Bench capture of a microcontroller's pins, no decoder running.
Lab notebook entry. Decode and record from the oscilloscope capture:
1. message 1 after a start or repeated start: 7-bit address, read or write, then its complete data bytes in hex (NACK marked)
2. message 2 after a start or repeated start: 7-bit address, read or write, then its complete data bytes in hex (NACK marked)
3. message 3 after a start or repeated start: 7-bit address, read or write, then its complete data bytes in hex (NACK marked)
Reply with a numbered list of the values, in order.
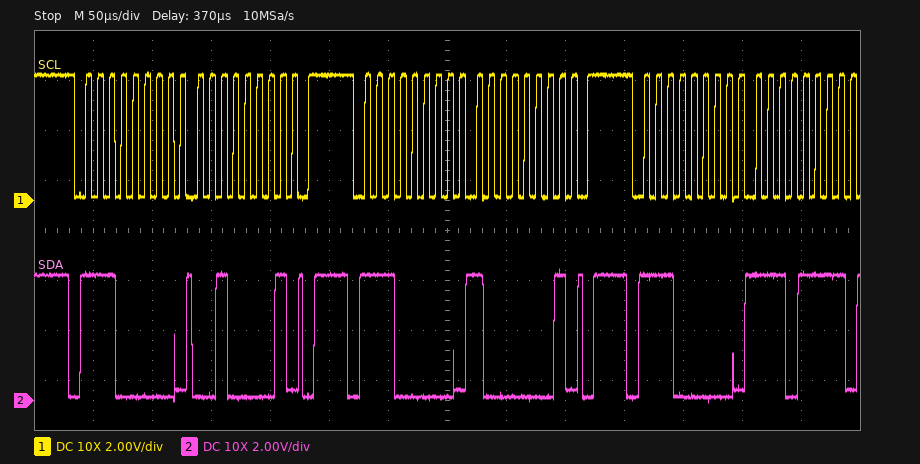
1. 0x70 write: 21
2. 0x70 write: 81
3. 0x70 write: EF
